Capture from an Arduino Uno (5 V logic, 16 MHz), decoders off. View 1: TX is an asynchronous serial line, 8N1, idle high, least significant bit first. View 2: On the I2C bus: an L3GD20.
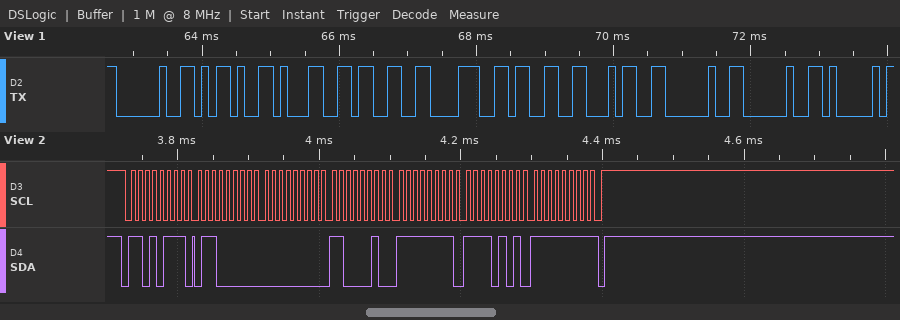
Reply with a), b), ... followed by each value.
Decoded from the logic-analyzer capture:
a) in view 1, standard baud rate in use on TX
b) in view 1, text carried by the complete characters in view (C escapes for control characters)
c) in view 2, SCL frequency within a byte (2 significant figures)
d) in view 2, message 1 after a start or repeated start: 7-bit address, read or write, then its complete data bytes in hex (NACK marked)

a) 9600 baud
b) " -13834  A"
c) 100 kHz
d) 0x6B read: 60 00 C2 FF F5 FF NACK
